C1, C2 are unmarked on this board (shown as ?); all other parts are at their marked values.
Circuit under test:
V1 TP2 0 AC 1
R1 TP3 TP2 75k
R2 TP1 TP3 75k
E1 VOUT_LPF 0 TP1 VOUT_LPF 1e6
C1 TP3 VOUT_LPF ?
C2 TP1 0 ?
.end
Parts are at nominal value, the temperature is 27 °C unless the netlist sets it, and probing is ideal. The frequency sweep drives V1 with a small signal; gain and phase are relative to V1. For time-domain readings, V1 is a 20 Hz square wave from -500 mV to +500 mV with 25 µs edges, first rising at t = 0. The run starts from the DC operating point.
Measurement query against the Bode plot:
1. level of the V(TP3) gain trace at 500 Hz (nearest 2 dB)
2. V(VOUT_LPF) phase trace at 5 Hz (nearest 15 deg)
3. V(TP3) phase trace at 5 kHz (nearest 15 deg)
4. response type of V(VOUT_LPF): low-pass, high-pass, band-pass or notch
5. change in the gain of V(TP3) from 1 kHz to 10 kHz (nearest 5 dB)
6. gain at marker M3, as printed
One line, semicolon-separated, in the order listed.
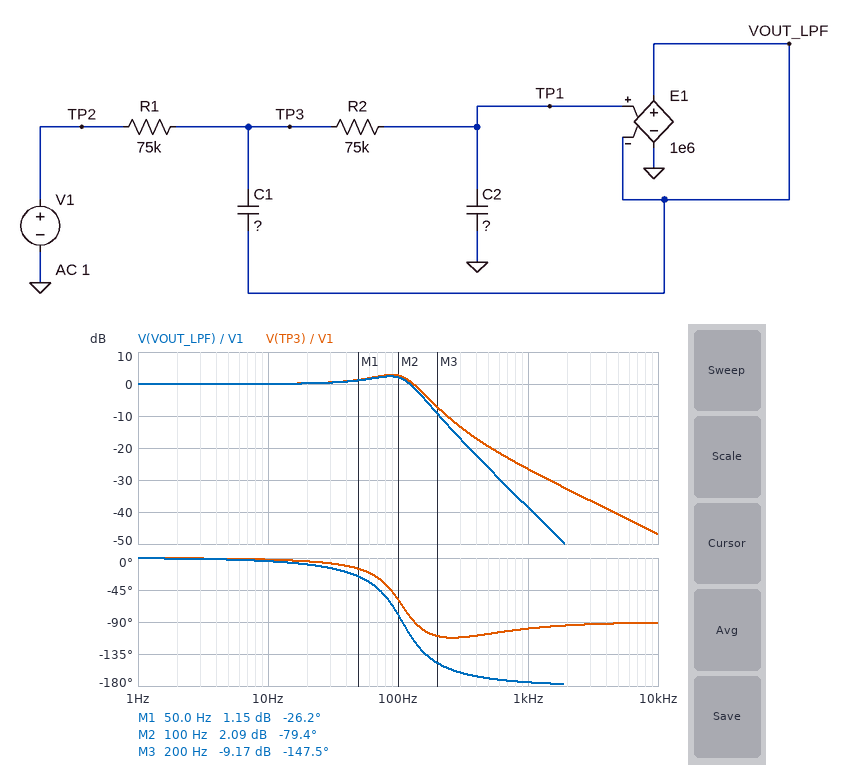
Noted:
-20 dB; 0 deg; -90 deg; low-pass; -20 dB; -9.17 dB
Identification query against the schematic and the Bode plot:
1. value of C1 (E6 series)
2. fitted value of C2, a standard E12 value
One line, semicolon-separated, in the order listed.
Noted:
47 nF; 8.2 nF
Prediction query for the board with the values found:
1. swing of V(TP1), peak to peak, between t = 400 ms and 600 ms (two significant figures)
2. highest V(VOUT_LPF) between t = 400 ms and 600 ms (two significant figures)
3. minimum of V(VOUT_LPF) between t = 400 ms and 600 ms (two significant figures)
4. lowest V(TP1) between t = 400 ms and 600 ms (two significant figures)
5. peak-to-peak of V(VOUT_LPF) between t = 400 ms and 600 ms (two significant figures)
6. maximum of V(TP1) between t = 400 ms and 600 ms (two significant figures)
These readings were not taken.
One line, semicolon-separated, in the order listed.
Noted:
1.5 V; 740 mV; -740 mV; -740 mV; 1.5 V; 740 mV
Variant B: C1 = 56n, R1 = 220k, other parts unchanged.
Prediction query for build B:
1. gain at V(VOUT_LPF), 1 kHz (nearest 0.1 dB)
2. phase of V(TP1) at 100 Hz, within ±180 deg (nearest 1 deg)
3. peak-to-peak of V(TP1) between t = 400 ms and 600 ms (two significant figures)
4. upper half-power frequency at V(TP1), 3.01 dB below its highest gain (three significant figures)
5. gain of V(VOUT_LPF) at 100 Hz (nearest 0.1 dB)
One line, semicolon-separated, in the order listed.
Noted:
-49.5 dB; -143 deg; 1.4 V; 68.5 Hz; -8.0 dB
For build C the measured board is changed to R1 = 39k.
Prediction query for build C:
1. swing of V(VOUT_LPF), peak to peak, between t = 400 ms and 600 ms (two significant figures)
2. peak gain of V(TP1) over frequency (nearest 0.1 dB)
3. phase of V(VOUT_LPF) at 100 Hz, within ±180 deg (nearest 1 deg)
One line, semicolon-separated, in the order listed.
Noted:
1.4 V; 2.0 dB; -47 deg
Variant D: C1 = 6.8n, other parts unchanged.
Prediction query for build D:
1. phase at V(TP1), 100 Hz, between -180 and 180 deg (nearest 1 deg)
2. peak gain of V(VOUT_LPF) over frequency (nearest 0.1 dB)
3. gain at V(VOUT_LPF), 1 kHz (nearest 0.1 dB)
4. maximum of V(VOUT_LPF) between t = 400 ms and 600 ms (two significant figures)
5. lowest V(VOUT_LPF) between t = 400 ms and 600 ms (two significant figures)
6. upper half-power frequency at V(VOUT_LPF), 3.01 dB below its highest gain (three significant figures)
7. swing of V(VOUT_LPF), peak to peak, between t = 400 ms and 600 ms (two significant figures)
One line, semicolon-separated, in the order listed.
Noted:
-41 deg; 0 dB; -22.8 dB; 500 mV; -500 mV; 160 Hz; 1.0 V
